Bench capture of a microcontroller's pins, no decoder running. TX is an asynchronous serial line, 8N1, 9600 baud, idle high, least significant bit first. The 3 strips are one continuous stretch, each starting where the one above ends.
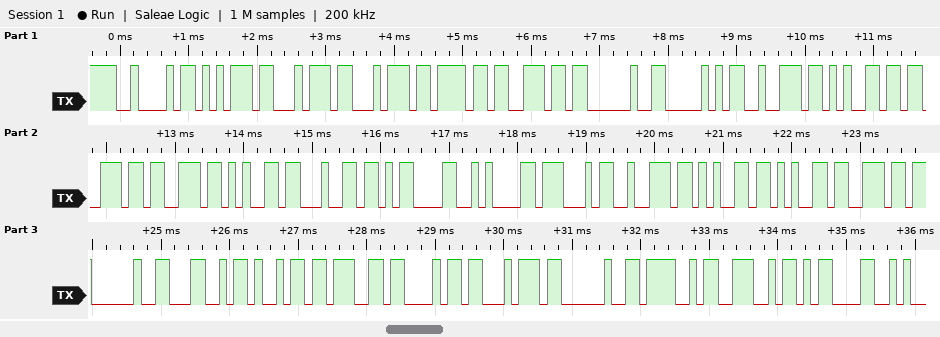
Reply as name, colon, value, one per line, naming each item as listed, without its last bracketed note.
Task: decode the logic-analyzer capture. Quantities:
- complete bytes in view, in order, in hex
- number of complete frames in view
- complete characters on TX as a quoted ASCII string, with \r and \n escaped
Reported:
complete bytes in view, in order, in hex: 42 75 74 74 6F 6E 20 50 72 65 73 73 65 64 0D 0A 47 72 65 65 6E 20 4C 69 67 68 74 20 4F 4E 0D
number of complete frames in view: 31
complete characters on TX as a quoted ASCII string, with \r and \n escaped: "Button Pressed\r\nGreen Light ON\r"
